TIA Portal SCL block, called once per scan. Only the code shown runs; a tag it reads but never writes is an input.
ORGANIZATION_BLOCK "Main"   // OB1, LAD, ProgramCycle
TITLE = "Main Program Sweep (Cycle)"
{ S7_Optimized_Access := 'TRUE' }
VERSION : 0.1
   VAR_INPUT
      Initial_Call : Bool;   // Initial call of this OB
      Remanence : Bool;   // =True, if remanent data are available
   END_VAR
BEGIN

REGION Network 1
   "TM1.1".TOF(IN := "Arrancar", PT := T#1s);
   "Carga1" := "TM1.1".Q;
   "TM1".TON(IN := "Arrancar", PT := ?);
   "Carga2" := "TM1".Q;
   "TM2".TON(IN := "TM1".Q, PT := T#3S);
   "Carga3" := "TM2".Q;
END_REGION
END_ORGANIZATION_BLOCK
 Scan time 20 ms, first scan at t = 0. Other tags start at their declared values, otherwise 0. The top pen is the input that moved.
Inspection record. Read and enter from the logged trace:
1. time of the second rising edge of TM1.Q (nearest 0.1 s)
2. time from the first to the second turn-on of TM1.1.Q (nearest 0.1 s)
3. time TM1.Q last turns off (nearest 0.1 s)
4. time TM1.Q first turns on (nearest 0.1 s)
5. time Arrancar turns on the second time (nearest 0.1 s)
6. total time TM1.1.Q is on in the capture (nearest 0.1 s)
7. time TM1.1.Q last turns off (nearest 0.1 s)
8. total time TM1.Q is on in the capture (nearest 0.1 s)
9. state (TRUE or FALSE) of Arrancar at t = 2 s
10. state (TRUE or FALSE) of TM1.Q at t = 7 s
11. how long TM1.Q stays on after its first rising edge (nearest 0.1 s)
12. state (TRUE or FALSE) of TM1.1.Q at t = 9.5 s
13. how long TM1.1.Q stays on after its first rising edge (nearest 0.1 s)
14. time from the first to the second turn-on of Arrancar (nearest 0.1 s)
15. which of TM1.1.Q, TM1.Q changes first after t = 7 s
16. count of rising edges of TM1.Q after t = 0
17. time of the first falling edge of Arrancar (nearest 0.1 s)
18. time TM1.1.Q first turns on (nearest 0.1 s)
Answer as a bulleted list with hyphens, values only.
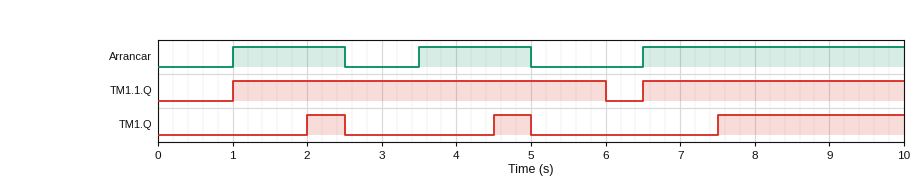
- 4.5 s
- 5.5 s
- 5.0 s
- 2.0 s
- 3.5 s
- 8.5 s
- 6.0 s
- 3.5 s
- TRUE
- FALSE
- 0.5 s
- TRUE
- 5.0 s
- 2.5 s
- TM1.Q
- 3
- 2.5 s
- 1.0 s
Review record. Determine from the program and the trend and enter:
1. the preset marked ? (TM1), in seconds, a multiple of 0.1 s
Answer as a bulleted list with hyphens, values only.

- 1.0 s
